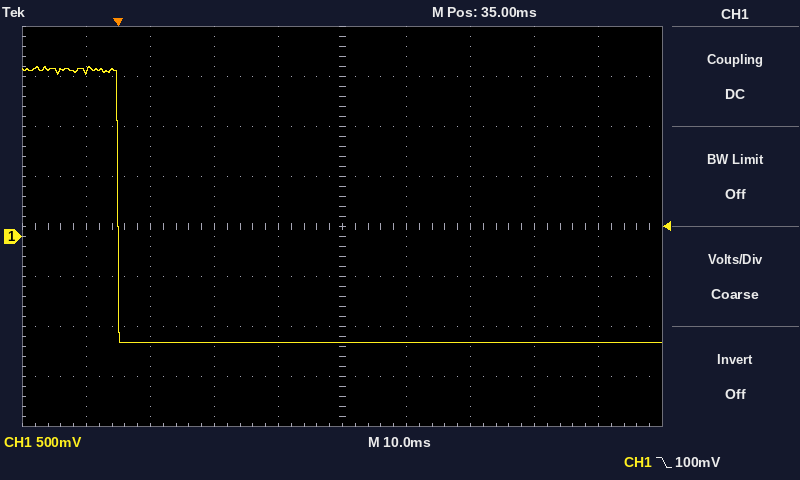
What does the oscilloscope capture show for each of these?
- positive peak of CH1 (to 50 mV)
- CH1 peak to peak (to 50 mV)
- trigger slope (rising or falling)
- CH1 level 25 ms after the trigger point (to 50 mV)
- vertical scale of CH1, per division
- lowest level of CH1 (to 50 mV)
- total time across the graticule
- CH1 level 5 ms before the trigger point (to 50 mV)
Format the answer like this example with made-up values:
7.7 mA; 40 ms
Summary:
1.70 V; 2.75 V; falling; -1.05 V; 500 mV; -1.05 V; 100 ms; 1.65 V
